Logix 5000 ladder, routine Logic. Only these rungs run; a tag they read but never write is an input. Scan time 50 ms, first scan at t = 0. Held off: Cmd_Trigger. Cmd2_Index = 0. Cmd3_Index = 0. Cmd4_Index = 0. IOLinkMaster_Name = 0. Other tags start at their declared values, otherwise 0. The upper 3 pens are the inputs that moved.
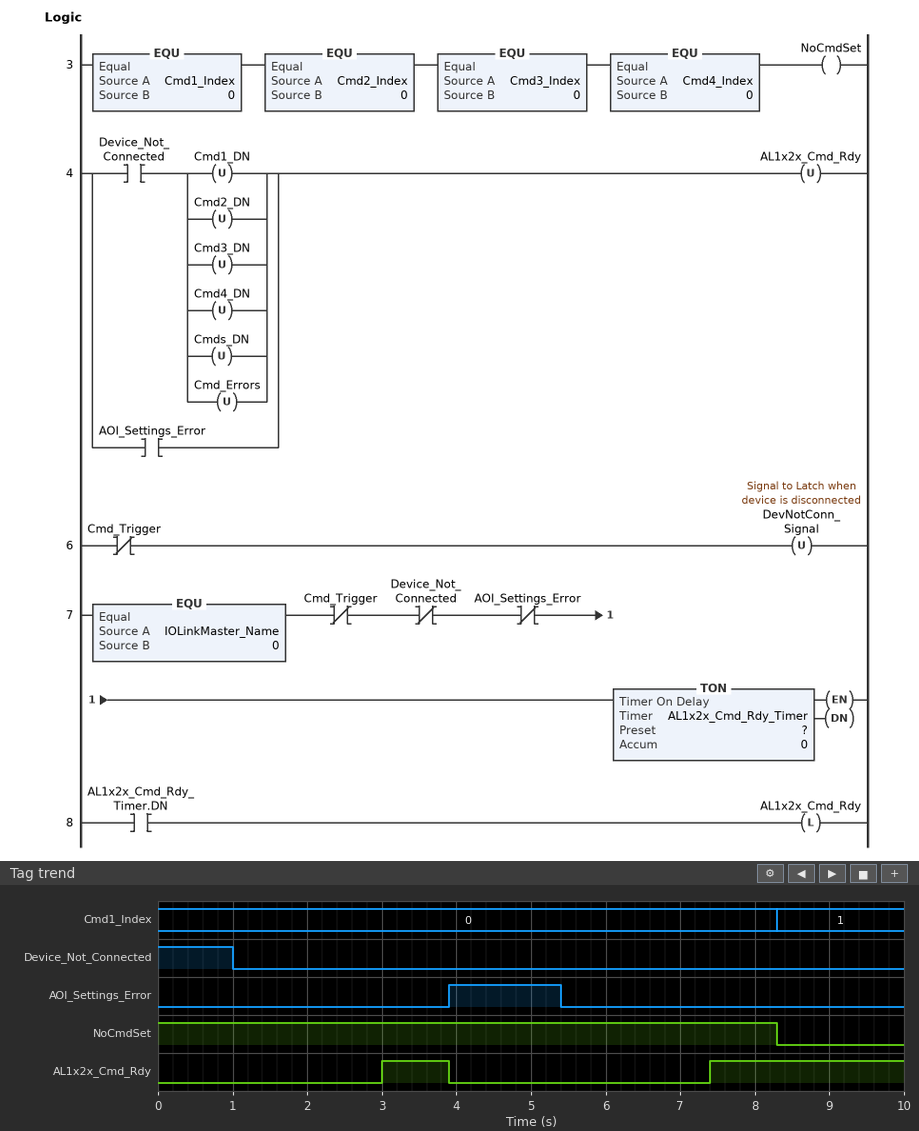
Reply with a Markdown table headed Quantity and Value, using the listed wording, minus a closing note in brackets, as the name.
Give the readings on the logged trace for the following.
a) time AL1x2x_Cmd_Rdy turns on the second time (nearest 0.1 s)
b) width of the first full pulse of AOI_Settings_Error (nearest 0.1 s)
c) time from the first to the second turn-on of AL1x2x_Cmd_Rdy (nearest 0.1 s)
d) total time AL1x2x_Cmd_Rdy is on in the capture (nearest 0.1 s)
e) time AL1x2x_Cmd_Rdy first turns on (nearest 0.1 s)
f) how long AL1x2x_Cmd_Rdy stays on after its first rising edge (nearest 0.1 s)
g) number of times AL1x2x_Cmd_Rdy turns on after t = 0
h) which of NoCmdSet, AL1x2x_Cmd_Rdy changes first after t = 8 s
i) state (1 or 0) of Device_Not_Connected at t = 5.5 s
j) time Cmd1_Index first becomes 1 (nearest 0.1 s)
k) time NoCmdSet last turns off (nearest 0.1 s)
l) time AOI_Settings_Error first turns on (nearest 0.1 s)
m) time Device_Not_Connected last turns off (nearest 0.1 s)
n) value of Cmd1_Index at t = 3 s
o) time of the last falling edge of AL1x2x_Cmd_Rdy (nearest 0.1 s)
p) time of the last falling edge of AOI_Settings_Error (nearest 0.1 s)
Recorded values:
| Quantity | Value |
|---|---|
| time AL1x2x_Cmd_Rdy turns on the second time | 7.4 s |
| width of the first full pulse of AOI_Settings_Error | 1.5 s |
| time from the first to the second turn-on of AL1x2x_Cmd_Rdy | 4.4 s |
| total time AL1x2x_Cmd_Rdy is on in the capture | 3.5 s |
| time AL1x2x_Cmd_Rdy first turns on | 3.0 s |
| how long AL1x2x_Cmd_Rdy stays on after its first rising edge | 0.9 s |
| number of times AL1x2x_Cmd_Rdy turns on after t = 0 | 2 |
| which of NoCmdSet, AL1x2x_Cmd_Rdy changes first after t = 8 s | NoCmdSet |
| state (1 or 0) of Device_Not_Connected at t = 5.5 s | 0 |
| time Cmd1_Index first becomes 1 | 8.3 s |
| time NoCmdSet last turns off | 8.3 s |
| time AOI_Settings_Error first turns on | 3.9 s |
| time Device_Not_Connected last turns off | 1.0 s |
| value of Cmd1_Index at t = 3 s | 0 |
| time of the last falling edge of AL1x2x_Cmd_Rdy | 3.9 s |
| time of the last falling edge of AOI_Settings_Error | 5.4 s |
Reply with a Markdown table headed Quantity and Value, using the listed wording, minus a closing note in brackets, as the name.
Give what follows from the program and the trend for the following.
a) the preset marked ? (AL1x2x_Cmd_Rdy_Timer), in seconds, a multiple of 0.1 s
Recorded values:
| Quantity | Value |
|---|---|
| the preset marked ? (AL1x2x_Cmd_Rdy_Timer), in seconds, a multiple of 0.1 s | 2.0 s |
